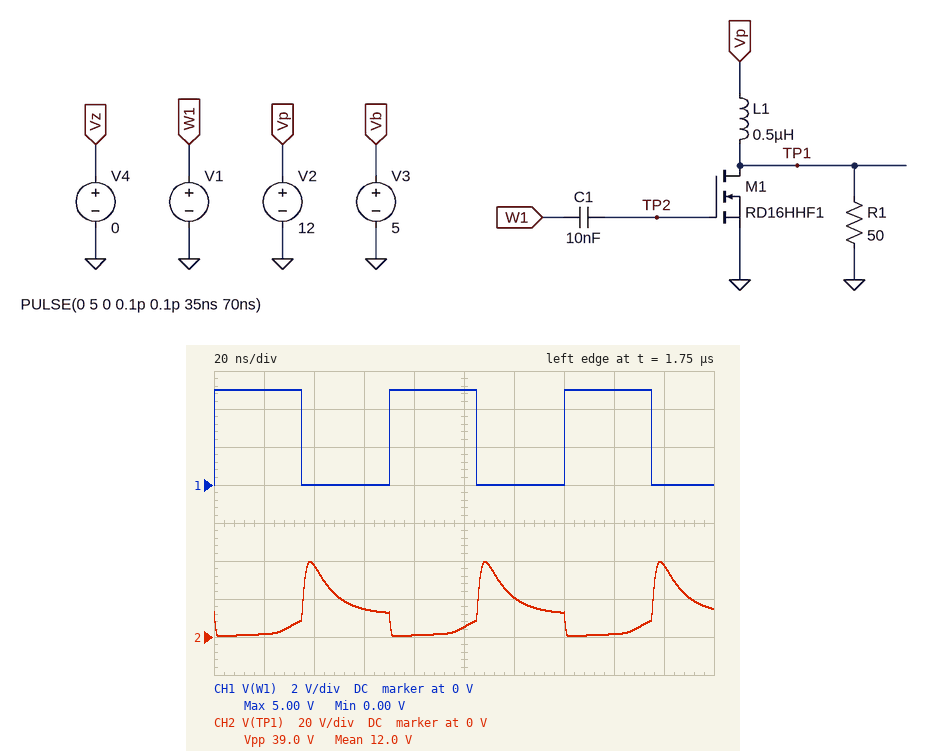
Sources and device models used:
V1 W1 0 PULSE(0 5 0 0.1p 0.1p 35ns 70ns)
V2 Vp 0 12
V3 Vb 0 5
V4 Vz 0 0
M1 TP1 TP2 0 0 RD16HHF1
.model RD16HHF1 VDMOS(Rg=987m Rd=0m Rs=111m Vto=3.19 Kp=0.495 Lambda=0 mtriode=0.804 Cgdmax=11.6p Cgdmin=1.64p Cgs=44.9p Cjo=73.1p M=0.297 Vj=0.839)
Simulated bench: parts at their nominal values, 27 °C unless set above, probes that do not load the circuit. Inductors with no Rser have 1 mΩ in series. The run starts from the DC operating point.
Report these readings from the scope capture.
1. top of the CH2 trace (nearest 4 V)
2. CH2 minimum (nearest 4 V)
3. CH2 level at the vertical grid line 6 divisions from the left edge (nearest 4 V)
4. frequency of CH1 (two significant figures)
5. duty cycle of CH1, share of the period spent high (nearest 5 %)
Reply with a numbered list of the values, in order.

1. 40 V
2. 0 V
3. 20 V
4. 14 MHz
5. 50 %
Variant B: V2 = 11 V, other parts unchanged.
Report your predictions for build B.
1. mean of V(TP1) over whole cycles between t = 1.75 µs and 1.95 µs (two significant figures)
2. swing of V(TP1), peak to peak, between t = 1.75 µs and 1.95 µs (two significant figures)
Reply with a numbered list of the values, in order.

1. 11 V
2. 37 V
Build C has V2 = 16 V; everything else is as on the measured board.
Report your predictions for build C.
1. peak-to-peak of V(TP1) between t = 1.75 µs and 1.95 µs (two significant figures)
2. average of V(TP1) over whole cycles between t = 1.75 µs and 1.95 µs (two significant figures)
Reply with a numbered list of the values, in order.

1. 44 V
2. 16 V
